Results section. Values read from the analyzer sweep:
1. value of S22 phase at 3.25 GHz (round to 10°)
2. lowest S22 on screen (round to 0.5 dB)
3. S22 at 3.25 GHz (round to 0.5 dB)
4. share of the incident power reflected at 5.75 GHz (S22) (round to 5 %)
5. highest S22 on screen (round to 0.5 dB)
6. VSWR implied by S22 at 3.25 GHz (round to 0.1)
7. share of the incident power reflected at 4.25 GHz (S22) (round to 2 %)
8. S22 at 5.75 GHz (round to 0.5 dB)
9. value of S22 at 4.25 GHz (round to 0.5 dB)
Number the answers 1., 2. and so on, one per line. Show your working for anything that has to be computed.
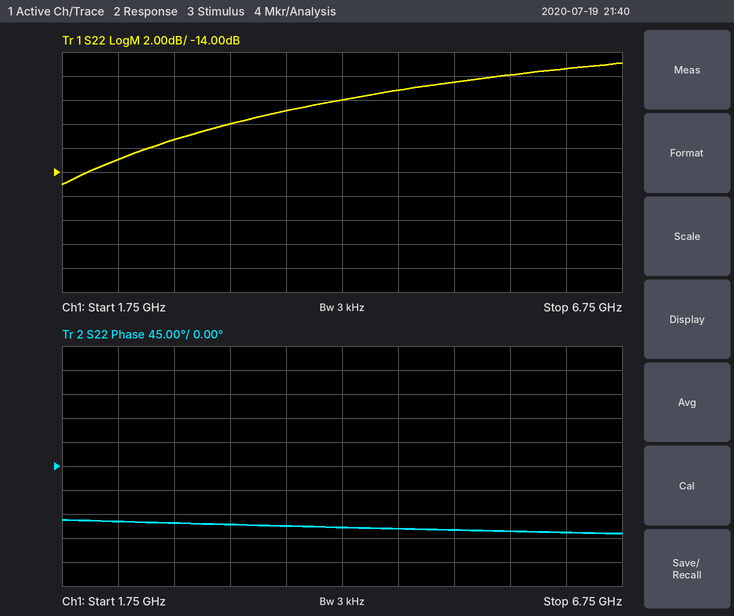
1. -110°
2. -15.0 dB
3. -10.0 dB
4. 10^(-6/10) ≈ 25 %
5. -5.0 dB
6. |Γ| = 10^(-10/20) = 0.3162; VSWR = (1 + 0.3162)/(1 − 0.3162) ≈ 1.9
7. 10^(-8/10) ≈ 16 %
8. -6.0 dB
9. -8.0 dB
